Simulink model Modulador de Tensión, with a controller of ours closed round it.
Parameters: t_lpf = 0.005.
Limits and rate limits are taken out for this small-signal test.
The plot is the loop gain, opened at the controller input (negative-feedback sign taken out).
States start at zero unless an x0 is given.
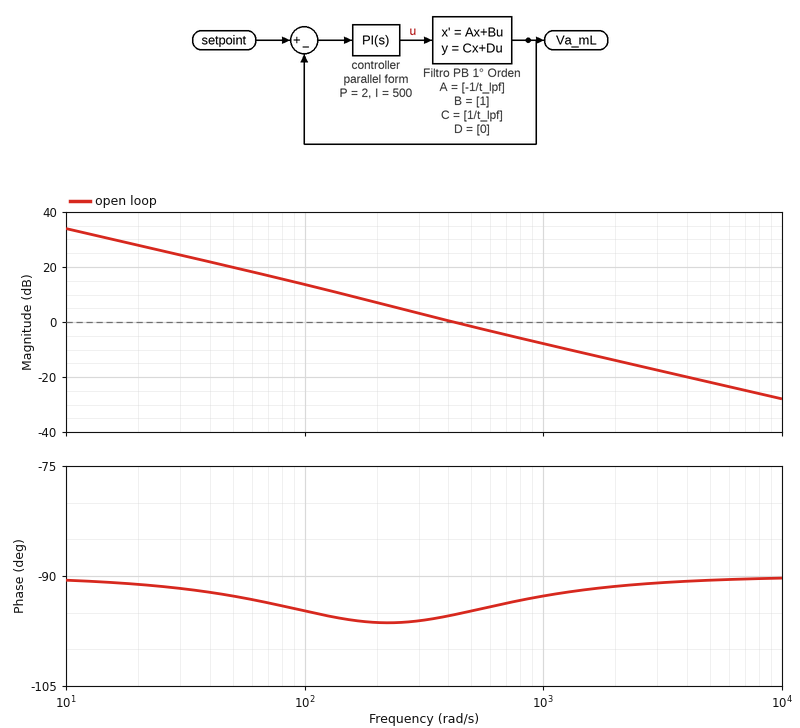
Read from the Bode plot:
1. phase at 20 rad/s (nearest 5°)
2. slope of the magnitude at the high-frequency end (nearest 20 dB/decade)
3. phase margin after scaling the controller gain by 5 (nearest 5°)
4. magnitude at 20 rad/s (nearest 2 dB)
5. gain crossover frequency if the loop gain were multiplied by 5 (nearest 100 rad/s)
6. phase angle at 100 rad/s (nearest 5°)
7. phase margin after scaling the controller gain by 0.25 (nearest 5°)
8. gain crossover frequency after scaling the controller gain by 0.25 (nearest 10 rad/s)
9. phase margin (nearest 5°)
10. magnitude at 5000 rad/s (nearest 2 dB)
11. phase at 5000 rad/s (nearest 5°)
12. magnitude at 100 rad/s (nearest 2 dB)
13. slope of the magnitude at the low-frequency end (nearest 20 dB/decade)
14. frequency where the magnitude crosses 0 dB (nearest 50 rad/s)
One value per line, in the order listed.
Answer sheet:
-90°
-20 dB/decade
90°
28 dB
2000 rad/s
-95°
85°
120 rad/s
85°
-22 dB
-90°
14 dB
-20 dB/decade
400 rad/s
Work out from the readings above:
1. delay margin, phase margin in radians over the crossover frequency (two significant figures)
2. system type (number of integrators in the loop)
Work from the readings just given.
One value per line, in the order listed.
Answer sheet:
0.0037 s
1
